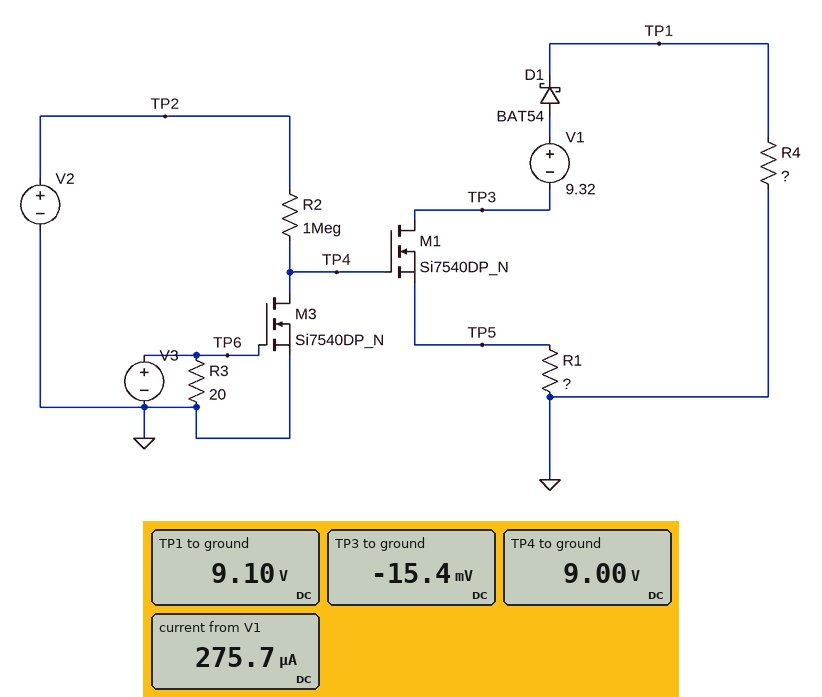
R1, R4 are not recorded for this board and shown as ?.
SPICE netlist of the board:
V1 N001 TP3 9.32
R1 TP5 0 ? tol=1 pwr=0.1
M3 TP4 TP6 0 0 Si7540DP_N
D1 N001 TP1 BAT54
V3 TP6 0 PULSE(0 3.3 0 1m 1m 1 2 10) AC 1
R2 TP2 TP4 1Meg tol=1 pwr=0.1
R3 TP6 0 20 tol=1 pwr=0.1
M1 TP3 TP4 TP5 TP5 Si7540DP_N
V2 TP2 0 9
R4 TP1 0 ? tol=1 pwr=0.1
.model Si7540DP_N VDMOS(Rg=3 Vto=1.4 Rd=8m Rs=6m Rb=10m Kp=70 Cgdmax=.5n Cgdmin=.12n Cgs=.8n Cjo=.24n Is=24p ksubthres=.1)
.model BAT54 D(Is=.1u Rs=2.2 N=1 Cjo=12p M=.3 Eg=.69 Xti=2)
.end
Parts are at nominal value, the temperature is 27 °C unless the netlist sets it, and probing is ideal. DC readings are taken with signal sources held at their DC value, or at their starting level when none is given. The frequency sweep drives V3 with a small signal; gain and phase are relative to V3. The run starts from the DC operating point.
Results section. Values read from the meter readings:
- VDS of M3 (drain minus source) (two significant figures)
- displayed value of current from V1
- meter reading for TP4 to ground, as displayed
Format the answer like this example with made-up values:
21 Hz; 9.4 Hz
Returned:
9.0 V; 275.7 µA; 9.00 V
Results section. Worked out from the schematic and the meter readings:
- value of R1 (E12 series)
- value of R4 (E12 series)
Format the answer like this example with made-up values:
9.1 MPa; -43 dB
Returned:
56 Ω; 33 kΩ
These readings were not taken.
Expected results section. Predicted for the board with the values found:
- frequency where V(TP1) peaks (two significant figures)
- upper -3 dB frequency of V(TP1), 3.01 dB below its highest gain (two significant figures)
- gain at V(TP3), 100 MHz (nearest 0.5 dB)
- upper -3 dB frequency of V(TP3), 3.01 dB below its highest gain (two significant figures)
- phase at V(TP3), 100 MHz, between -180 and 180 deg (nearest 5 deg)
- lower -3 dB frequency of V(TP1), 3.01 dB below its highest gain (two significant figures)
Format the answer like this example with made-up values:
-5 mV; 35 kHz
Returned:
31 MHz; 90 MHz; -9.5 dB; 90 MHz; -50 deg; 11 MHz
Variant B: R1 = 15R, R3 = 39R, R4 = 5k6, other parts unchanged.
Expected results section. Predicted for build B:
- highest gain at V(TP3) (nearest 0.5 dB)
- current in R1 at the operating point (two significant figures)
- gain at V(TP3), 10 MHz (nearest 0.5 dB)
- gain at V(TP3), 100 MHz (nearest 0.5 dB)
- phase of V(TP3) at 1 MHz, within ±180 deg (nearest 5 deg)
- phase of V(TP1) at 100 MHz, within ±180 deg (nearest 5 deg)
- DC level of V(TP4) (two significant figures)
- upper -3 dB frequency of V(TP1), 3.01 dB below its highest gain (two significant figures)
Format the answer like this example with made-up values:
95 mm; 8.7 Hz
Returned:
-10.5 dB; 1.6 mA; -19.5 dB; -12.0 dB; 90 deg; -30 deg; 9.0 V; 140 MHz
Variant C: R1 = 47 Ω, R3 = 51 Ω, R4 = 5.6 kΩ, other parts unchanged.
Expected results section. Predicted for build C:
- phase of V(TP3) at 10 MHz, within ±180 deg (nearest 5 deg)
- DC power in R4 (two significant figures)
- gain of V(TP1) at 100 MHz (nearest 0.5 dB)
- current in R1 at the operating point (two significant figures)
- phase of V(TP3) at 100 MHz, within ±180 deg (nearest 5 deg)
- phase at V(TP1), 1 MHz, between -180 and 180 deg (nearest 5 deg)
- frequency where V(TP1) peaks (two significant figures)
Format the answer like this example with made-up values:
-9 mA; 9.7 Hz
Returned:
50 deg; 14 mW; -10.0 dB; 1.6 mA; -45 deg; 85 deg; 34 MHz
